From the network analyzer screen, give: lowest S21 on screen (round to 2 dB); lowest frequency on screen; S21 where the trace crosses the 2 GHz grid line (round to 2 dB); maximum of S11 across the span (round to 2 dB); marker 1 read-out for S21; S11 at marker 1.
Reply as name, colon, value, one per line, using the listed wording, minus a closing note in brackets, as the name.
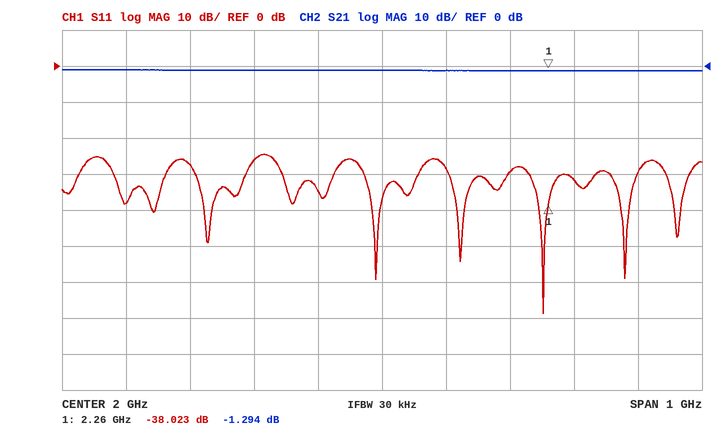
lowest S21 on screen: -2 dB
lowest frequency on screen: 1.5 GHz
S21 where the trace crosses the 2 GHz grid line: -2 dB
maximum of S11 across the span: -24 dB
marker 1 read-out for S21: -1.294 dB
S11 at marker 1: -38.023 dB
